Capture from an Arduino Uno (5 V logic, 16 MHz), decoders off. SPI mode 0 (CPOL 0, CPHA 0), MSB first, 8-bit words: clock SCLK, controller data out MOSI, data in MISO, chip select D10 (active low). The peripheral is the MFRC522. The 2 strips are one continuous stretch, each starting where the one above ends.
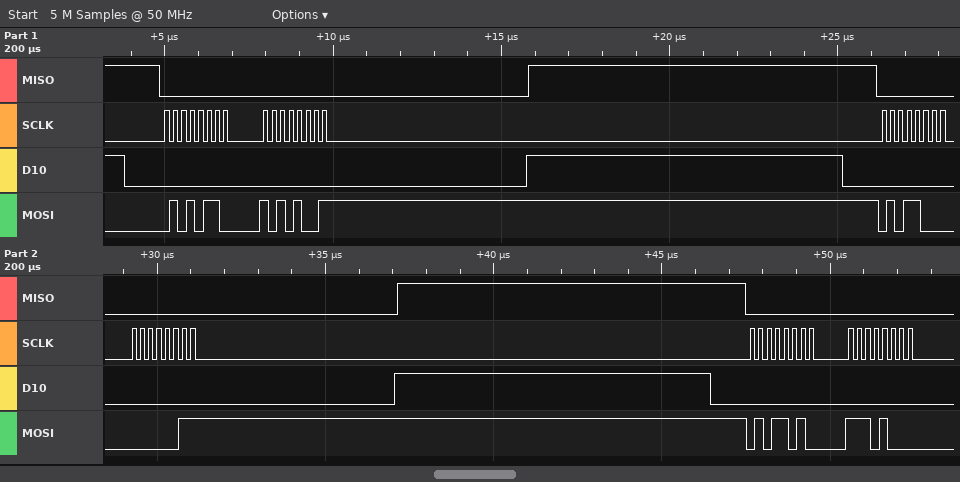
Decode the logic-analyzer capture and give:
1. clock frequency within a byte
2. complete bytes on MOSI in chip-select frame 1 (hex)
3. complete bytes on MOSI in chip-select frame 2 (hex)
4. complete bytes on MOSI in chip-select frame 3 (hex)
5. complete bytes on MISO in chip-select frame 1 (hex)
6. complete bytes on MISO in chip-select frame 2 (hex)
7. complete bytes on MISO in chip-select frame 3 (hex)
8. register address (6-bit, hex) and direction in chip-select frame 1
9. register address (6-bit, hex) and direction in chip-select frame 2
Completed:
4 MHz
56 A9
58 03
5A E8
00 00
00 00
00 00
0x2B write
0x2C write
